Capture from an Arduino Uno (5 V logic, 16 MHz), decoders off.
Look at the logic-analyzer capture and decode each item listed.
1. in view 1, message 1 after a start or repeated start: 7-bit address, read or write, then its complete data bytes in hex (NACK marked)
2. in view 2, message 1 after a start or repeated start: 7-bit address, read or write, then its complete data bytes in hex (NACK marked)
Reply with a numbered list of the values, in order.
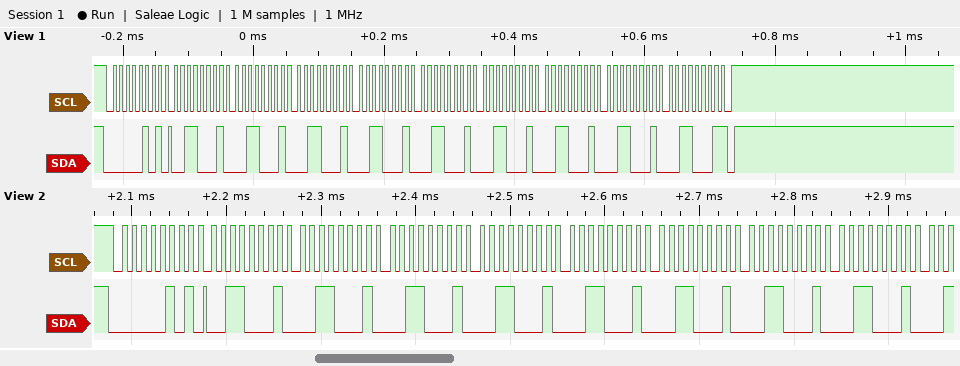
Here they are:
1. 0x02 read: 31 31 31 31 31 31 31 31 31 NACK
2. 0x02 read: 31 31 31 31 31 31 31 31
